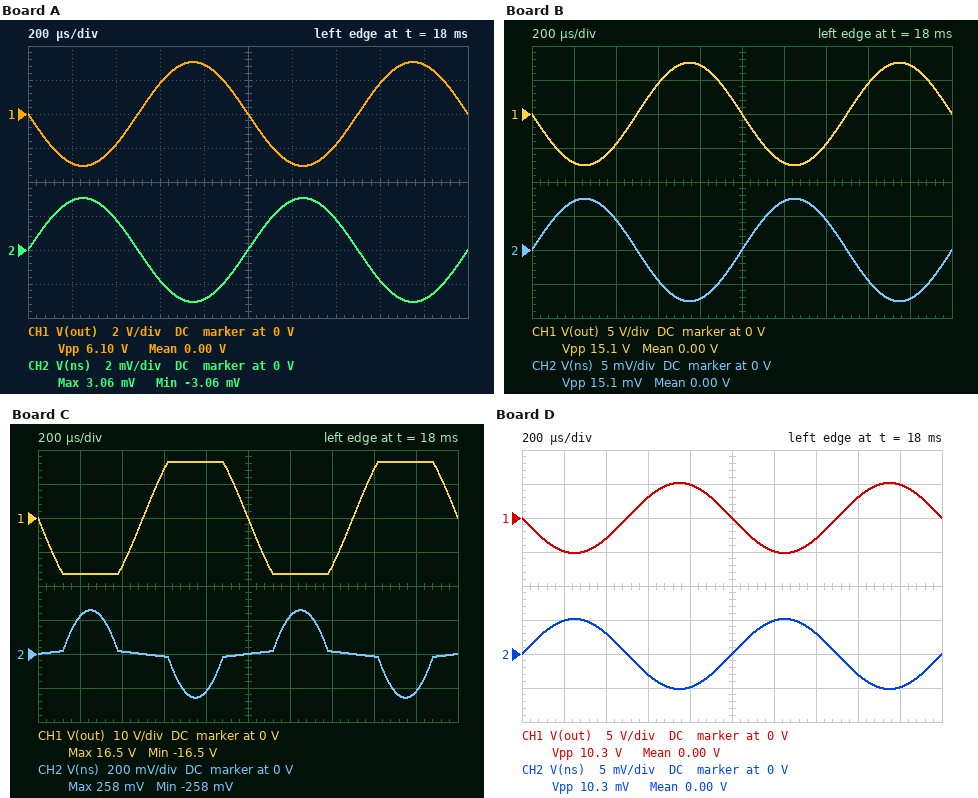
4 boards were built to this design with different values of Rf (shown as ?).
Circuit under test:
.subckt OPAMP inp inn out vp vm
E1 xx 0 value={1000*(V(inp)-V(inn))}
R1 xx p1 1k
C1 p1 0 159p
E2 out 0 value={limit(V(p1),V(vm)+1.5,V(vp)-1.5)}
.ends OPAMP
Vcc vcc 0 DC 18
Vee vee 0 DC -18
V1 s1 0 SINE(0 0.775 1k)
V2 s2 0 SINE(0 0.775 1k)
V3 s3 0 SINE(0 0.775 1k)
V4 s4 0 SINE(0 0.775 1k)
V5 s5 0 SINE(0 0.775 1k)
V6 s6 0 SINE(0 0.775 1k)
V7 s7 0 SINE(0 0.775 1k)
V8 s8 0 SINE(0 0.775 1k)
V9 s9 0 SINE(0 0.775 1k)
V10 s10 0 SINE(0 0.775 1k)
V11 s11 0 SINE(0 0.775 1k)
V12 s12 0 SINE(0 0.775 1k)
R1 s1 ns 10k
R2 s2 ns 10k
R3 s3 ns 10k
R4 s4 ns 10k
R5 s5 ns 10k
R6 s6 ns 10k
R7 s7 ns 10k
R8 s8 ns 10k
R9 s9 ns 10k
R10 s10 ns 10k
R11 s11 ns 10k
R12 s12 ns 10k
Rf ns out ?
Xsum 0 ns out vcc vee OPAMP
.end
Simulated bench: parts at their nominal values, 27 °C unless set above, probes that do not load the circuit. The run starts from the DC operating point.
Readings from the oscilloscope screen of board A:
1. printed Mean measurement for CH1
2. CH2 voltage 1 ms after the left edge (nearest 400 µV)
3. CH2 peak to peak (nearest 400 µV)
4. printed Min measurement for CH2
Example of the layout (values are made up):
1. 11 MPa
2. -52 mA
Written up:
1. 0.00 V
2. 0 V
3. 6.0 mV
4. -3.06 mV
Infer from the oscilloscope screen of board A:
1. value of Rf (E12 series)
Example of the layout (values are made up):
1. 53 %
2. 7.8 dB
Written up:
1. 3.3 kΩ
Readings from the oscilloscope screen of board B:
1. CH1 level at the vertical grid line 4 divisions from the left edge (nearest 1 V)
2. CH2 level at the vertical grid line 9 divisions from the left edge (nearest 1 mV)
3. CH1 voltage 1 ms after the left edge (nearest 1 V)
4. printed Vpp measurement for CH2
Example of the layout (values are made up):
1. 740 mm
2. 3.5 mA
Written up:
1. 7 V
2. -7 mV
3. 0 V
4. 15.1 mV
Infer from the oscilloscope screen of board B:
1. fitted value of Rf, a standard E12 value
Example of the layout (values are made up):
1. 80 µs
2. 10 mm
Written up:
1. 8.2 kΩ
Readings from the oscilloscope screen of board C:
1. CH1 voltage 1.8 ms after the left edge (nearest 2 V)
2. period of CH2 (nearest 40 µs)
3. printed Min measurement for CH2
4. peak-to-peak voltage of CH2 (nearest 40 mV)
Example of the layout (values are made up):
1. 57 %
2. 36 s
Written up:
1. 16 V
2. 1.00 ms
3. -258 mV
4. 520 mV
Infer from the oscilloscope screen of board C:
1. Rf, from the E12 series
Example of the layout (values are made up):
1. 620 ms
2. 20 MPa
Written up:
1. 27 kΩ
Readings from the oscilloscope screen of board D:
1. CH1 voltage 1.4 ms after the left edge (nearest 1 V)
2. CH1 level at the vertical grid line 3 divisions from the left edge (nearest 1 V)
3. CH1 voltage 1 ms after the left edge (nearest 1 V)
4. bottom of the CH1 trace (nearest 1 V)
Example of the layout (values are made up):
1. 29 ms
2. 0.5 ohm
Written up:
1. -3 V
2. 3 V
3. 0 V
4. -5 V
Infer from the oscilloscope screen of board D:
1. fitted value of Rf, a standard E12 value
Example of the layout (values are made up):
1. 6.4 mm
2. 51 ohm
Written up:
1. 5.6 kΩ
